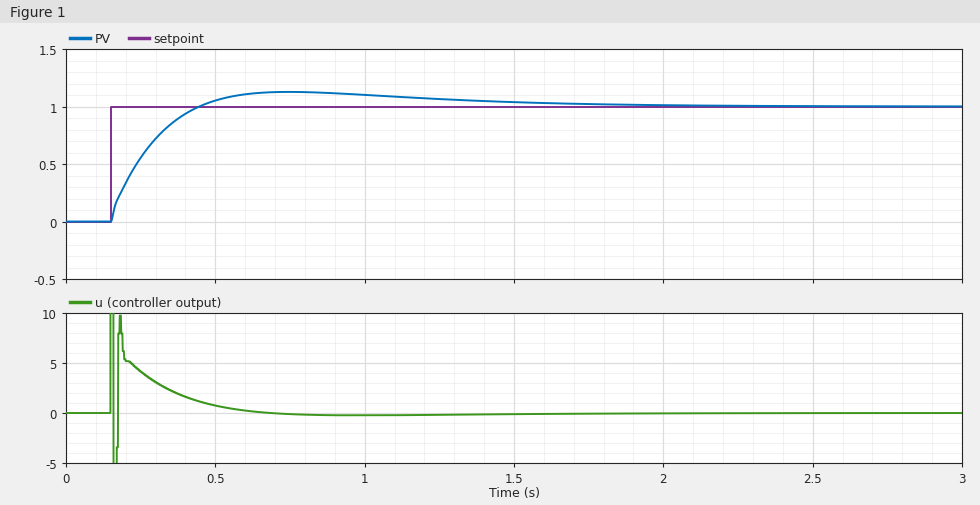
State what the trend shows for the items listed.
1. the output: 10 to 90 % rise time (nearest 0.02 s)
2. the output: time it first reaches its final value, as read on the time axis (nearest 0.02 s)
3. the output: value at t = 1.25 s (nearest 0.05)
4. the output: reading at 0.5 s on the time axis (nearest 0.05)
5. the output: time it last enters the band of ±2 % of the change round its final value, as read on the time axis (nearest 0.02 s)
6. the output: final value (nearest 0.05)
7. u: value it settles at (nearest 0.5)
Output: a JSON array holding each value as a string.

["0.22 s", "0.44 s", "1.05", "1.05", "1.78 s", "1.00", "0.0"]
